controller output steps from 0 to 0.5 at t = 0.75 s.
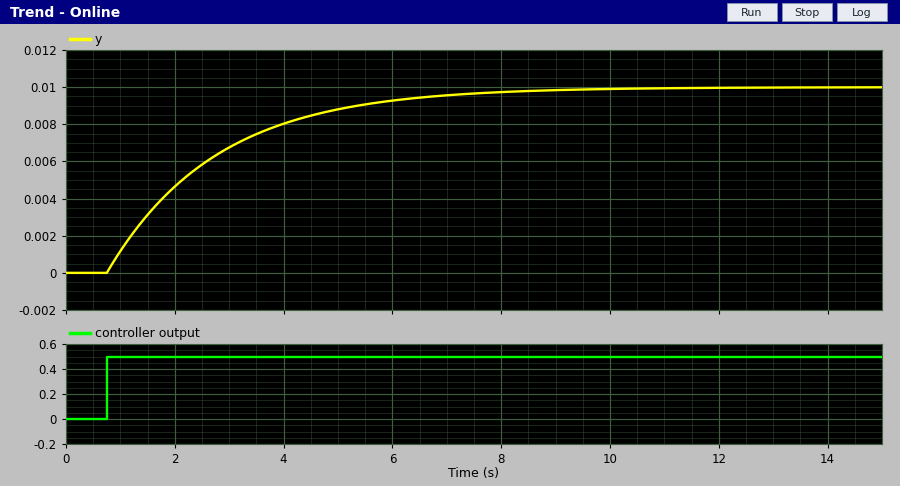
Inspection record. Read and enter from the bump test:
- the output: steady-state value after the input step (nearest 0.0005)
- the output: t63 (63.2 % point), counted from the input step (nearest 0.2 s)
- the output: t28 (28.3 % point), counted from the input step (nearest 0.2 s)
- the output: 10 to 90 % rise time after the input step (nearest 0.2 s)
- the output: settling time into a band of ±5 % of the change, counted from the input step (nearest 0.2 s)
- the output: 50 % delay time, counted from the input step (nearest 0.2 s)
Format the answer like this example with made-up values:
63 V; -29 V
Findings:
0.0100; 2.0 s; 0.6 s; 4.4 s; 6.0 s; 1.4 s
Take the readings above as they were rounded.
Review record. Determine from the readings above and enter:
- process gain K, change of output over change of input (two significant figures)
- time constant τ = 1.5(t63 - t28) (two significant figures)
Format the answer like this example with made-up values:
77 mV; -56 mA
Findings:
0.020; 2.1 s
